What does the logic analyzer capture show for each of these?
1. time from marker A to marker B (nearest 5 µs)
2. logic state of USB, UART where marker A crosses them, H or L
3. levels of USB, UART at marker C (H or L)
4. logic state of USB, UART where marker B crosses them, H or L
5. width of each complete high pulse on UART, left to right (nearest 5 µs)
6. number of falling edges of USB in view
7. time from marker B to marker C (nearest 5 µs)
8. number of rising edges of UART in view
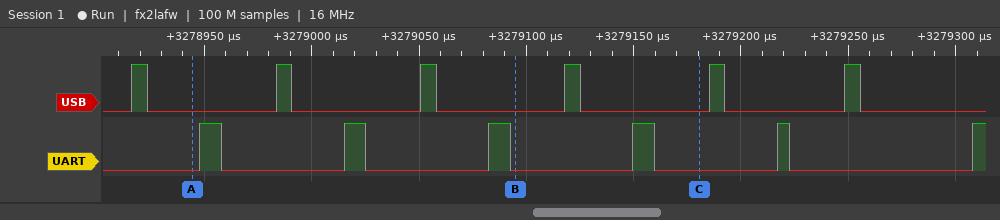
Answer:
150 µs
USB=L, UART=L
USB=L, UART=L
USB=L, UART=L
10 µs, 10 µs, 10 µs, 10 µs, 5 µs
6
85 µs
6
